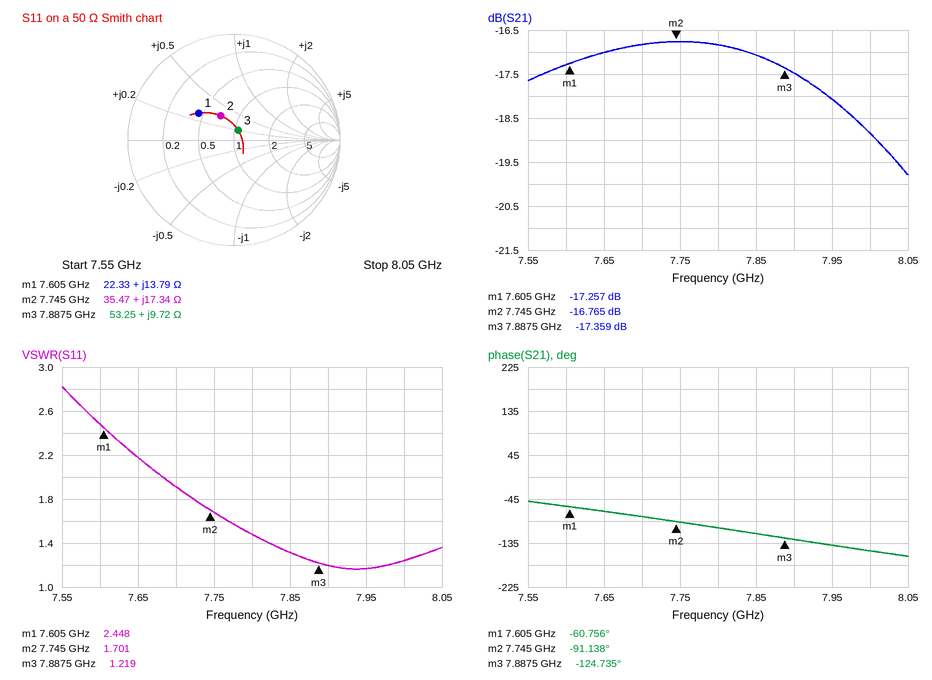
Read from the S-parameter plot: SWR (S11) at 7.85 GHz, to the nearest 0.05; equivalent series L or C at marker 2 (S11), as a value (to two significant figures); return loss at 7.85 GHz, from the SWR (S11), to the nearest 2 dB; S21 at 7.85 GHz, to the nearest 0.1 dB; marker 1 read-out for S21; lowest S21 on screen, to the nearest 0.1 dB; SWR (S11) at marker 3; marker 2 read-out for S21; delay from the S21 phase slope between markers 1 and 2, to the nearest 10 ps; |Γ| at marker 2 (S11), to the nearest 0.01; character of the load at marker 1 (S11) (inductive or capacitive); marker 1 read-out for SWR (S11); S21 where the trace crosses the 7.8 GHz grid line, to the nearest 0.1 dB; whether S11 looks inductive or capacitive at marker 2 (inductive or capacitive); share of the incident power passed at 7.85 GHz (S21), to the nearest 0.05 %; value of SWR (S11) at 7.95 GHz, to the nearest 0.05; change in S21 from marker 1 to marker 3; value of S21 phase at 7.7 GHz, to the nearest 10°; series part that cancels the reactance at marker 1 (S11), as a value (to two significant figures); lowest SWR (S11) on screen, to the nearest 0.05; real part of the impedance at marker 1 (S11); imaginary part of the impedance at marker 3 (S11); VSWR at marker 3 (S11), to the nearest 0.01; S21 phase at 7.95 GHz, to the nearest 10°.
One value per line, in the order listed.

1.30
360 pH
18 dB
-17.1 dB
-17.257 dB
-19.8 dB
1.219
-16.765 dB
600 ps
0.26
inductive
2.448
-16.8 dB
inductive
1.95 %
1.15
-0.102 dB
-80°
1.5 pF
1.15
22.33 Ω
+9.72 Ω
1.22
-140°
